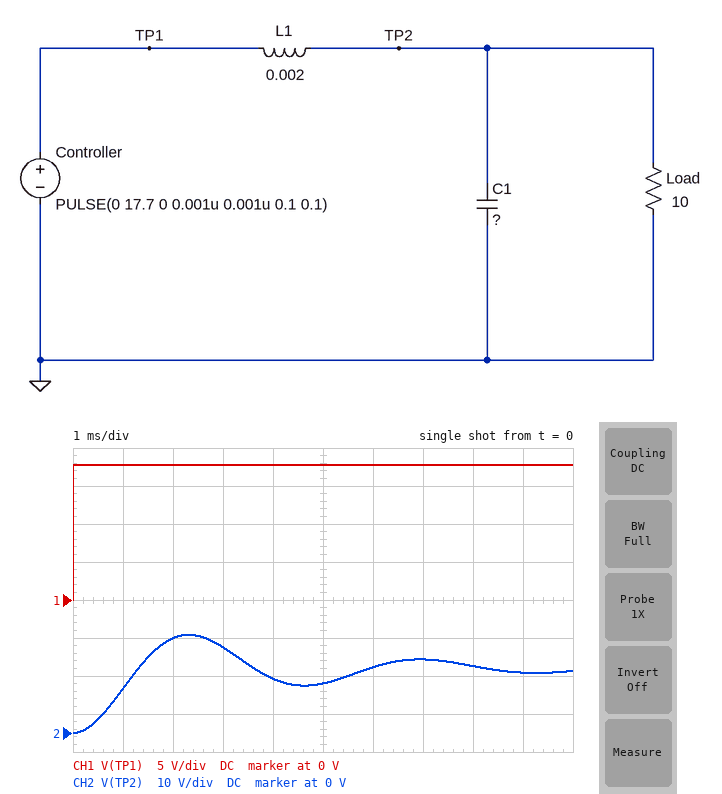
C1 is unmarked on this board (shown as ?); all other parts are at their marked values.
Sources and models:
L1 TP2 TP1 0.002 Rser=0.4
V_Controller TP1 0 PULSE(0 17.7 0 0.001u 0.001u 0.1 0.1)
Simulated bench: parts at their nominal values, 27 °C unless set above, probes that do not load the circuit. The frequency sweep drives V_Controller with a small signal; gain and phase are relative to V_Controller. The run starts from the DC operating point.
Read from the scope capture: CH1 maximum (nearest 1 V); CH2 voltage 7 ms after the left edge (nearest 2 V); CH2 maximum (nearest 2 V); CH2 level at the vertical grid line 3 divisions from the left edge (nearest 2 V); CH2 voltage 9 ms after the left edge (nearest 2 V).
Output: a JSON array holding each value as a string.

["18 V", "20 V", "26 V", "22 V", "16 V"]
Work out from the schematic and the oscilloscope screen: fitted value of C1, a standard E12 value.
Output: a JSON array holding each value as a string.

["270 µF"]
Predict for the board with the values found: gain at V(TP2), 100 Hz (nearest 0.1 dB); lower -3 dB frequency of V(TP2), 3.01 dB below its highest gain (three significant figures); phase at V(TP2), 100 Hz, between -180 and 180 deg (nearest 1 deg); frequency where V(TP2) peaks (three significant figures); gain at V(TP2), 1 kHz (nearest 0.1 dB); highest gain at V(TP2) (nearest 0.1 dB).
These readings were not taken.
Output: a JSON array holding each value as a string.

["1.4 dB", "158 Hz", "-13 deg", "211 Hz", "-26.2 dB", "7.6 dB"]
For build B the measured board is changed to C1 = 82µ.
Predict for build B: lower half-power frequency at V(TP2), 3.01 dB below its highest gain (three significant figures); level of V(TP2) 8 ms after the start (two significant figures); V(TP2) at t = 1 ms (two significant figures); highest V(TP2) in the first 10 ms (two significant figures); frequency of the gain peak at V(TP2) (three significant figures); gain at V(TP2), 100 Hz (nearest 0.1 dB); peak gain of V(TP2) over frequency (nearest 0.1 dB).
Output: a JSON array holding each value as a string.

["220 Hz", "17 V", "22 V", "24 V", "368 Hz", "0.1 dB", "5.0 dB"]
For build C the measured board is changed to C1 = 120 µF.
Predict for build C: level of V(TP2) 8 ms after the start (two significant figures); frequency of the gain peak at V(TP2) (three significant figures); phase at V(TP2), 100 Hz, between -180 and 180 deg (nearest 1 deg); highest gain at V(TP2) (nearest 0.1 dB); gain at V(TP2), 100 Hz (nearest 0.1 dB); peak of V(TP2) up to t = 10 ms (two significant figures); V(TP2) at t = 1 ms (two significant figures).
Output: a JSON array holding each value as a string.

["17 V", "310 Hz", "-9 deg", "6.0 dB", "0.4 dB", "25 V", "19 V"]
